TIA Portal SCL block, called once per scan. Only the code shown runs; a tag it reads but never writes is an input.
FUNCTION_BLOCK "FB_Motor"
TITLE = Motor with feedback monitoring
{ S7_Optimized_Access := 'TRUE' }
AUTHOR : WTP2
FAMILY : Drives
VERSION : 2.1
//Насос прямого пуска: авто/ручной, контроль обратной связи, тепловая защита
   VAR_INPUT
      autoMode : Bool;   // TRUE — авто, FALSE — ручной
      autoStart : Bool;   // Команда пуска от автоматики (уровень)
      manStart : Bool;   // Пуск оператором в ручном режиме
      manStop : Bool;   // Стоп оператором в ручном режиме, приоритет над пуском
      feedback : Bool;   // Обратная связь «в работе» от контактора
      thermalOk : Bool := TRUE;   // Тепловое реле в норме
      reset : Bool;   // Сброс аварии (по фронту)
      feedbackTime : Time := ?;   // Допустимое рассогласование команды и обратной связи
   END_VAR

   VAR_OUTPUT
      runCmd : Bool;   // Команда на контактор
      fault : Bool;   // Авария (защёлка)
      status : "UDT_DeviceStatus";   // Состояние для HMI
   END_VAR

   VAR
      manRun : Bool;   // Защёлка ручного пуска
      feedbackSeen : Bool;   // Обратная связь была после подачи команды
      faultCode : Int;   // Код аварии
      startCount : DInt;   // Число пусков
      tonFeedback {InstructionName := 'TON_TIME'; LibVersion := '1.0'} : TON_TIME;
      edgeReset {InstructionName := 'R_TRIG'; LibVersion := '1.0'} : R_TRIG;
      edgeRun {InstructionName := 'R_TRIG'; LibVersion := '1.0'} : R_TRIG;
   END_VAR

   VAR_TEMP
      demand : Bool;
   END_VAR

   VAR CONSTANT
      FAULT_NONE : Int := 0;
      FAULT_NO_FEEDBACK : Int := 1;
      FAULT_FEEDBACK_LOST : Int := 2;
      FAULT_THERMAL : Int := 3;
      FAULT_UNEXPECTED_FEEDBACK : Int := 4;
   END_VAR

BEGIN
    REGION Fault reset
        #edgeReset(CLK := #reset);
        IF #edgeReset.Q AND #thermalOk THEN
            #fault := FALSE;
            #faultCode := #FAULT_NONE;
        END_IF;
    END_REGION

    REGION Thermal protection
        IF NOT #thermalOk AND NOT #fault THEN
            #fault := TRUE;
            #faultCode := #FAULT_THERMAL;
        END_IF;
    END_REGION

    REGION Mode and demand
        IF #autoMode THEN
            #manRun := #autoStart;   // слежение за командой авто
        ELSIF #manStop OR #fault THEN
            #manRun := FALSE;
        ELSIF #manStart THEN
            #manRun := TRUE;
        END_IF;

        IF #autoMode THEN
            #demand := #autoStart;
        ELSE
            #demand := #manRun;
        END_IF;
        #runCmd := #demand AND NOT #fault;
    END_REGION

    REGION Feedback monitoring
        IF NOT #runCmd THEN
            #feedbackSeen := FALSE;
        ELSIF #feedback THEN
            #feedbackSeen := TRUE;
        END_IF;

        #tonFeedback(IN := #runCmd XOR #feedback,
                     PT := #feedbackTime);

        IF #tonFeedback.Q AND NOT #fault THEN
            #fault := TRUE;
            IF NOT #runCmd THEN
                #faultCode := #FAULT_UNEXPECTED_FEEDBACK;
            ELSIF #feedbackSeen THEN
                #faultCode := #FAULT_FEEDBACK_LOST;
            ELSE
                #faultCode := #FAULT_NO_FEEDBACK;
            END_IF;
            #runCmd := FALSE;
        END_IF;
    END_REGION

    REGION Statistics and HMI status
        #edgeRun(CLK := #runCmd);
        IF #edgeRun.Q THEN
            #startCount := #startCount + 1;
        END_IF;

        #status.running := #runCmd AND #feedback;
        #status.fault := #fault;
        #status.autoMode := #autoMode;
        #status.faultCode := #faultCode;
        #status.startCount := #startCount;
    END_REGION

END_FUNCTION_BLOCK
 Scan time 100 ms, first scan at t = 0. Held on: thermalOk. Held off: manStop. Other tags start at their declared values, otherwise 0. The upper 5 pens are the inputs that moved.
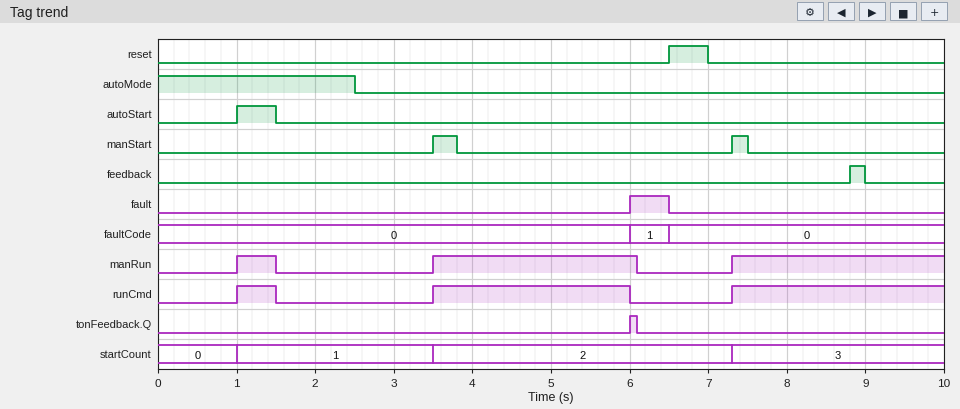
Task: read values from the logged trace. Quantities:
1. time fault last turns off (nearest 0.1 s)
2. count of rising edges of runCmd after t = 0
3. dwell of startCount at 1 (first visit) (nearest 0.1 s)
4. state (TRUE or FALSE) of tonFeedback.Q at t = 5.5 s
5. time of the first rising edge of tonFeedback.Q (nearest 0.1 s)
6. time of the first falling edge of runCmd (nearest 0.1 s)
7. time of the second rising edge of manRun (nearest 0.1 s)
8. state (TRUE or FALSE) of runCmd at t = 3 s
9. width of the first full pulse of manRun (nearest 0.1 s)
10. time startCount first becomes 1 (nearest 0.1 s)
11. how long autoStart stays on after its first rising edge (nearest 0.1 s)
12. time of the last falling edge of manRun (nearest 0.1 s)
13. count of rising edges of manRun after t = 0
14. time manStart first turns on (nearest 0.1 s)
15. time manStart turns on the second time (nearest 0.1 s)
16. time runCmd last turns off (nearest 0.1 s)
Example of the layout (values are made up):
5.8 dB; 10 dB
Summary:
6.5 s; 3; 2.5 s; FALSE; 6.0 s; 1.5 s; 3.5 s; FALSE; 0.5 s; 1.0 s; 0.5 s; 6.1 s; 3; 3.5 s; 7.3 s; 6.0 s
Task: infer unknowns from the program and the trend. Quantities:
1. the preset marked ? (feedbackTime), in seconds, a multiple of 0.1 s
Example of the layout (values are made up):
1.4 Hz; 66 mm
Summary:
2.5 s
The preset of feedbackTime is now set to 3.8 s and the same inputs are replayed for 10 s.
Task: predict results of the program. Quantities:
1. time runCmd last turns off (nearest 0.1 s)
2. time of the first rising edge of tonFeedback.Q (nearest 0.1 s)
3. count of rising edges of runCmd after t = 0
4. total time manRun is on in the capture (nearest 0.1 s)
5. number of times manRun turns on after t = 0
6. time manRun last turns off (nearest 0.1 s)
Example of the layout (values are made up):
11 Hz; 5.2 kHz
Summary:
7.3 s; 7.3 s; 2; 4.4 s; 2; 7.4 s
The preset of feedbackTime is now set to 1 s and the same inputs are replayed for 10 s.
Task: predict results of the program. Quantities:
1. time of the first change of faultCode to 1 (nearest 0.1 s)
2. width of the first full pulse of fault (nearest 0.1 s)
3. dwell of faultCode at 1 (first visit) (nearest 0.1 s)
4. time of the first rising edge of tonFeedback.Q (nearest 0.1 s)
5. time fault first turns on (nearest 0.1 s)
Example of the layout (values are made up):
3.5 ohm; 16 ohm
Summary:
4.5 s; 2.0 s; 2.0 s; 4.5 s; 4.5 s
